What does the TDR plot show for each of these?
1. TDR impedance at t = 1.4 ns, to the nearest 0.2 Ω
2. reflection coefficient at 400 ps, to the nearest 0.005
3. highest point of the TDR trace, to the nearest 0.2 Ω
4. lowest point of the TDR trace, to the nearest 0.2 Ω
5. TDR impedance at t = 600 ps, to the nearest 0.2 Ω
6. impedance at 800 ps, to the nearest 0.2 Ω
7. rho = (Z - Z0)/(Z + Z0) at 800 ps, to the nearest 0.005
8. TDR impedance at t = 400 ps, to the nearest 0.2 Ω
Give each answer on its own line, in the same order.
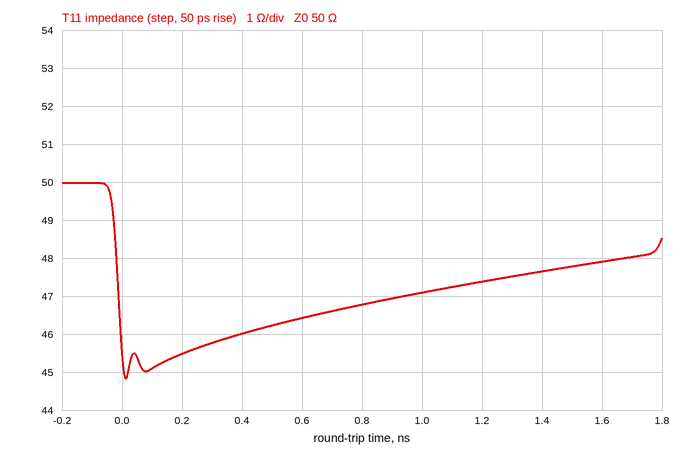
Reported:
47.6 Ω
-0.040
50.0 Ω
44.8 Ω
46.4 Ω
46.8 Ω
-0.035
46.0 Ω
